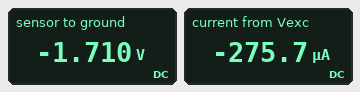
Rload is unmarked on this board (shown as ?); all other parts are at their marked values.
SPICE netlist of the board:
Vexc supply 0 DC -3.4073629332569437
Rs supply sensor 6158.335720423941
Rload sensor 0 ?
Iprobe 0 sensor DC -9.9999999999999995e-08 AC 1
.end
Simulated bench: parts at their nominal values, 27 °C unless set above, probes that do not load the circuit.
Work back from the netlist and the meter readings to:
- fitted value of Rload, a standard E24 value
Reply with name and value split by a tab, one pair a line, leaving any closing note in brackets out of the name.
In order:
fitted value of Rload, a standard E24 value	6.2 kΩ
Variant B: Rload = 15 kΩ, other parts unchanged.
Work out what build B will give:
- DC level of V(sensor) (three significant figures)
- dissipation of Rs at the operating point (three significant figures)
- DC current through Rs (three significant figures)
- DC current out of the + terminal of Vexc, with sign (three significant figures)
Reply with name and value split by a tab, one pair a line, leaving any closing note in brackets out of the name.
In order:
DC level of V(sensor)	-2.42 V
dissipation of Rs at the operating point	160 µW
DC current through Rs	161 µA
DC current out of the + terminal of Vexc, with sign	-161 µA
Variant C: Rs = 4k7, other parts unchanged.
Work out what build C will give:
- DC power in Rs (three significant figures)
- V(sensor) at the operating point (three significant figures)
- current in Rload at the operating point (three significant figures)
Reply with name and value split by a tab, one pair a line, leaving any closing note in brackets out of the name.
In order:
DC power in Rs	459 µW
V(sensor) at the operating point	-1.94 V
current in Rload at the operating point	313 µA
